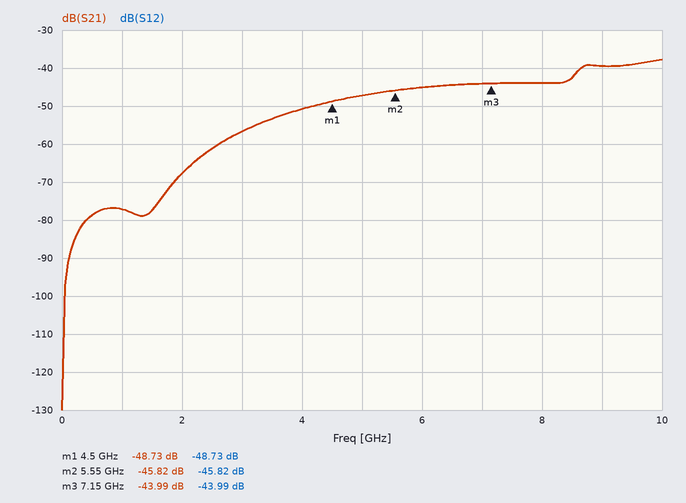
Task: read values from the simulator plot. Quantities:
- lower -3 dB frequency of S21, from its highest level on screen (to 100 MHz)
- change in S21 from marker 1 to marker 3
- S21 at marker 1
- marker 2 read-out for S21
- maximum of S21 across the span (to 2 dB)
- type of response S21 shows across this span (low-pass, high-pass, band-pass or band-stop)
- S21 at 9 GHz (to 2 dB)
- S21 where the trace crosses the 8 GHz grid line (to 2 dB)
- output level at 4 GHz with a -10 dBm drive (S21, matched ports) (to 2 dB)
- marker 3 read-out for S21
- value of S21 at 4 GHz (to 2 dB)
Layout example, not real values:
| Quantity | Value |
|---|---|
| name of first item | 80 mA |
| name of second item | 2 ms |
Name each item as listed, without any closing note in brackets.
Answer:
| Quantity | Value |
|---|---|
| lower -3 dB frequency of S21, from its highest level on screen | 8.6 GHz |
| change in S21 from marker 1 to marker 3 | 4.74 dB |
| S21 at marker 1 | -48.73 dB |
| marker 2 read-out for S21 | -45.82 dB |
| maximum of S21 across the span | -38 dB |
| type of response S21 shows across this span | high-pass |
| S21 at 9 GHz | -40 dB |
| S21 where the trace crosses the 8 GHz grid line | -44 dB |
| output level at 4 GHz with a -10 dBm drive (S21, matched ports) | -60 dBm |
| marker 3 read-out for S21 | -43.99 dB |
| value of S21 at 4 GHz | -50 dB |
